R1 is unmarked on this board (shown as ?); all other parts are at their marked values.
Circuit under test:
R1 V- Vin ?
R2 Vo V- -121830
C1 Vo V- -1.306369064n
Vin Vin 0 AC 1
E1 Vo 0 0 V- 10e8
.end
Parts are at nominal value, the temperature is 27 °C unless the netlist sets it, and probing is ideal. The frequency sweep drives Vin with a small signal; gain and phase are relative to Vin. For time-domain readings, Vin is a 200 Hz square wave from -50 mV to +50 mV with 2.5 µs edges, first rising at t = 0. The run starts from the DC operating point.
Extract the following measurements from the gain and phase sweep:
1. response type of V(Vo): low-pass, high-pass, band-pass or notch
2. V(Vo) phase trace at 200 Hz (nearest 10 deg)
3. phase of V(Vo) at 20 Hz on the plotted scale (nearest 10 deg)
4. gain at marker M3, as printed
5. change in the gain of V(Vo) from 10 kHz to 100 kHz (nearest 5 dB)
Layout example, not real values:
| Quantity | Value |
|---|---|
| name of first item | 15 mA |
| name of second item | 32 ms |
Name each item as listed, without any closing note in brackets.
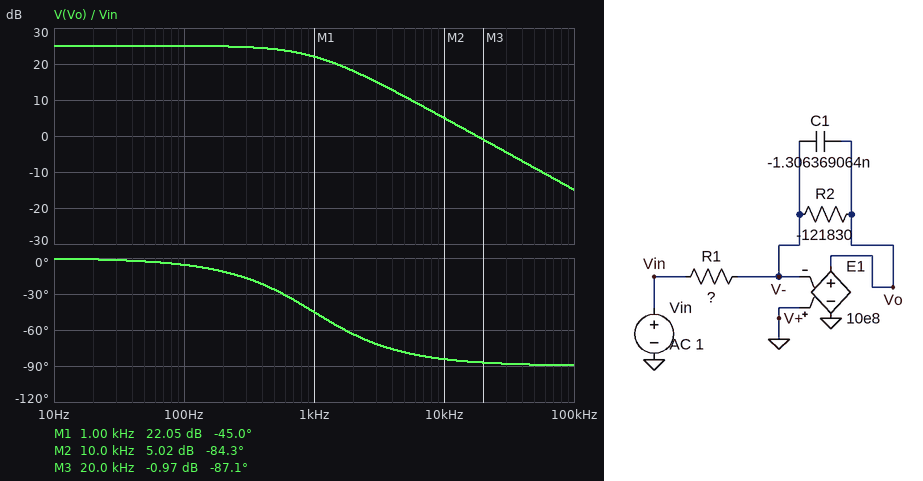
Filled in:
| Quantity | Value |
|---|---|
| response type of V(Vo): low-pass, high-pass, band-pass or notch | low-pass |
| V(Vo) phase trace at 200 Hz | -10 deg |
| phase of V(Vo) at 20 Hz on the plotted scale | 0 deg |
| gain at marker M3, as printed | -0.97 dB |
| change in the gain of V(Vo) from 10 kHz to 100 kHz | -20 dB |
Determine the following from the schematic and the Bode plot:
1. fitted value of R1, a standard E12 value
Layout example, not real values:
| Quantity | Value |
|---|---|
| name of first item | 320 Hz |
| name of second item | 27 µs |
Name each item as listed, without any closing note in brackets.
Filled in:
| Quantity | Value |
|---|---|
| fitted value of R1, a standard E12 value | 6.8 kΩ |
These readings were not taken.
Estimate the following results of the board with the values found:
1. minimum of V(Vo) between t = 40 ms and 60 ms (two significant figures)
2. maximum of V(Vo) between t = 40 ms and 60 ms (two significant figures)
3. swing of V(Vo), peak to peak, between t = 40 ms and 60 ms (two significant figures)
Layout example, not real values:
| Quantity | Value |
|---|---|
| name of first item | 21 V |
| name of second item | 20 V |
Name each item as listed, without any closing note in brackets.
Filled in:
| Quantity | Value |
|---|---|
| minimum of V(Vo) between t = 40 ms and 60 ms | -900 mV |
| maximum of V(Vo) between t = 40 ms and 60 ms | 900 mV |
| swing of V(Vo), peak to peak, between t = 40 ms and 60 ms | 1.8 V |
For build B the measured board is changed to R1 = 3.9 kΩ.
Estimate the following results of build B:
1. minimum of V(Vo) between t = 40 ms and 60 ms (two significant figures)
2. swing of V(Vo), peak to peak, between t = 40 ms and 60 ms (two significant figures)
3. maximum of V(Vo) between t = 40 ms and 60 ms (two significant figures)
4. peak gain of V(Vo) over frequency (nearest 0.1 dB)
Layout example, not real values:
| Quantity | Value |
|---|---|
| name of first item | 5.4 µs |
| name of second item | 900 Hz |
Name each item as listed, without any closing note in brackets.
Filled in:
| Quantity | Value |
|---|---|
| minimum of V(Vo) between t = 40 ms and 60 ms | -1.6 V |
| swing of V(Vo), peak to peak, between t = 40 ms and 60 ms | 3.1 V |
| maximum of V(Vo) between t = 40 ms and 60 ms | 1.6 V |
| peak gain of V(Vo) over frequency | 29.9 dB |
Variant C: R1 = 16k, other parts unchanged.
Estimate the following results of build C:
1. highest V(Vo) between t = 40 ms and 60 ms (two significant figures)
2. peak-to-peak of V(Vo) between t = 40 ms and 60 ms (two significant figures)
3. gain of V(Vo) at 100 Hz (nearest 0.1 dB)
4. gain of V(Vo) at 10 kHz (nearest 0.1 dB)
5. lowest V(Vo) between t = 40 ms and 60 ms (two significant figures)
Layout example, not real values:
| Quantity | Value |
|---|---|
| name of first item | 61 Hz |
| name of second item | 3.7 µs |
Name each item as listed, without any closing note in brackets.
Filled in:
| Quantity | Value |
|---|---|
| highest V(Vo) between t = 40 ms and 60 ms | 380 mV |
| peak-to-peak of V(Vo) between t = 40 ms and 60 ms | 760 mV |
| gain of V(Vo) at 100 Hz | 17.6 dB |
| gain of V(Vo) at 10 kHz | -2.4 dB |
| lowest V(Vo) between t = 40 ms and 60 ms | -380 mV |
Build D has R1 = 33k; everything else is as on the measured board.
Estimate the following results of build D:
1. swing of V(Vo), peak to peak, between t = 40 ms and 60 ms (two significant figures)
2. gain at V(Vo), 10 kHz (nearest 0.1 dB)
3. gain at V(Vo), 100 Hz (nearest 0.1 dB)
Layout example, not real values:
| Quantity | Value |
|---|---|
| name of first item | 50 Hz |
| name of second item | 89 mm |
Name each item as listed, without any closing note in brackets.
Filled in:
| Quantity | Value |
|---|---|
| swing of V(Vo), peak to peak, between t = 40 ms and 60 ms | 370 mV |
| gain at V(Vo), 10 kHz | -8.7 dB |
| gain at V(Vo), 100 Hz | 11.3 dB |
